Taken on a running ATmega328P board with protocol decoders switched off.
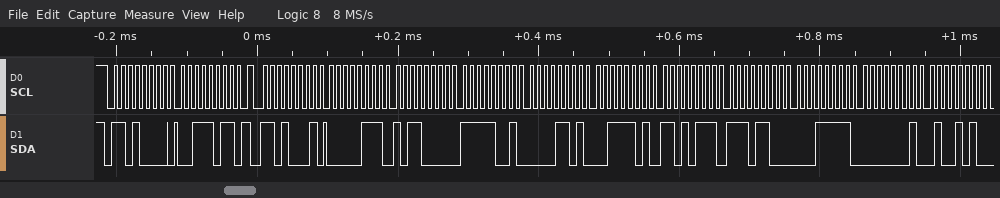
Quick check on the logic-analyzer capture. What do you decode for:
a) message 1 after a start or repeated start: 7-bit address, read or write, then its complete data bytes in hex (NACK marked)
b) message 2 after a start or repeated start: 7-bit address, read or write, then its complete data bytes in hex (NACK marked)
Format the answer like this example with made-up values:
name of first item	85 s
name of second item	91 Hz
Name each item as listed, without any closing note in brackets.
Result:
message 1 after a start or repeated start: 7-bit address, read or write, then its complete data bytes in hex	0x68 write: 3B
message 2 after a start or repeated start: 7-bit address, read or write, then its complete data bytes in hex	0x68 read: 07 B0 F9 0D 3D D7 EC 1F 01 4A
